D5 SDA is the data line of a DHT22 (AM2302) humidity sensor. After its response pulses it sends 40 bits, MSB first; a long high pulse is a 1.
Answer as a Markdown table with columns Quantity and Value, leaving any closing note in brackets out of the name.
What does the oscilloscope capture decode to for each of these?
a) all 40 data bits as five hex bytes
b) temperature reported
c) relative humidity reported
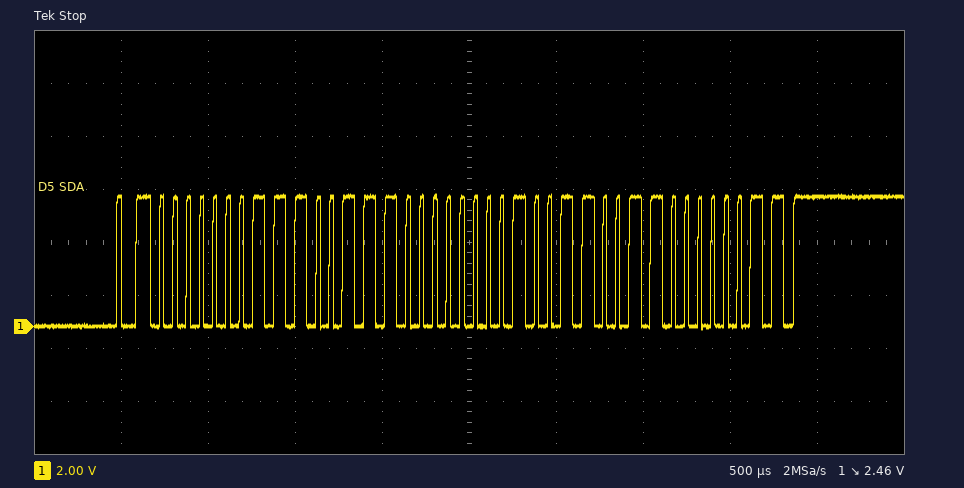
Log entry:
| Quantity | Value |
|---|---|
| all 40 data bits as five hex bytes | 01 CE 01 33 03 |
| temperature reported | 30.7 °C |
| relative humidity reported | 46.2 % |
